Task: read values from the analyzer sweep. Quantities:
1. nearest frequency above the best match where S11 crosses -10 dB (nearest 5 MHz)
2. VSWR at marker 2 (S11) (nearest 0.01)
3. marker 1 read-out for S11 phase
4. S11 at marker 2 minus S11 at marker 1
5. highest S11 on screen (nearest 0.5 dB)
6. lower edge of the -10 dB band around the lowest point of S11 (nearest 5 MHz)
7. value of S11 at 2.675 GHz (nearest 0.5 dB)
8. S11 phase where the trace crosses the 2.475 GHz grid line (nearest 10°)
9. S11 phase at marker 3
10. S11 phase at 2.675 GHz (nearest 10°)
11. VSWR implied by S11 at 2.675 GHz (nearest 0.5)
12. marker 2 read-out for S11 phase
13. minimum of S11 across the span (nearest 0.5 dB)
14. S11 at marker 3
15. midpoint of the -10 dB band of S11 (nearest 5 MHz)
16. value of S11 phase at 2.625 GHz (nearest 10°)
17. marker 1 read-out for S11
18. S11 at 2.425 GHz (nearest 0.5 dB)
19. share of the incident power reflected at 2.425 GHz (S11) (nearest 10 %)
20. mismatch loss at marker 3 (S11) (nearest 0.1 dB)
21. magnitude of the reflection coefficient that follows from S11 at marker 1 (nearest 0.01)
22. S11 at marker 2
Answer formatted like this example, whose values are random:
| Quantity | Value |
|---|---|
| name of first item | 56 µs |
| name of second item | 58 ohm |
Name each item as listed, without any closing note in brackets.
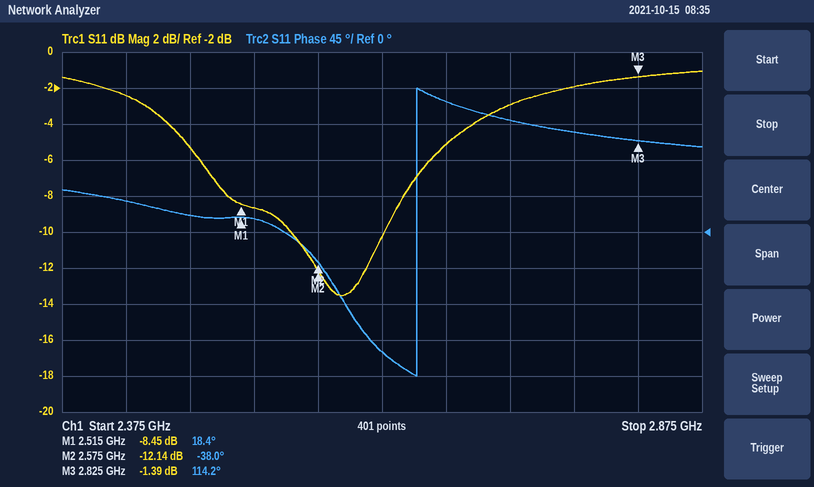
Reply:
| Quantity | Value |
|---|---|
| nearest frequency above the best match where S11 crosses -10 dB | 2.625 GHz |
| VSWR at marker 2 (S11) | 1.66 |
| marker 1 read-out for S11 phase | 18.4° |
| S11 at marker 2 minus S11 at marker 1 | -3.69 dB |
| highest S11 on screen | -1.0 dB |
| lower edge of the -10 dB band around the lowest point of S11 | 2.555 GHz |
| value of S11 at 2.675 GHz | -5.0 dB |
| S11 phase where the trace crosses the 2.475 GHz grid line | 20° |
| S11 phase at marker 3 | 114.2° |
| S11 phase at 2.675 GHz | 160° |
| VSWR implied by S11 at 2.675 GHz | 3.5 |
| marker 2 read-out for S11 phase | -38.0° |
| minimum of S11 across the span | -13.5 dB |
| S11 at marker 3 | -1.39 dB |
| midpoint of the -10 dB band of S11 | 2.590 GHz |
| value of S11 phase at 2.625 GHz | -150° |
| marker 1 read-out for S11 | -8.45 dB |
| S11 at 2.425 GHz | -2.5 dB |
| share of the incident power reflected at 2.425 GHz (S11) | 60 % |
| mismatch loss at marker 3 (S11) | 5.6 dB |
| magnitude of the reflection coefficient that follows from S11 at marker 1 | 0.38 |
| S11 at marker 2 | -12.14 dB |
